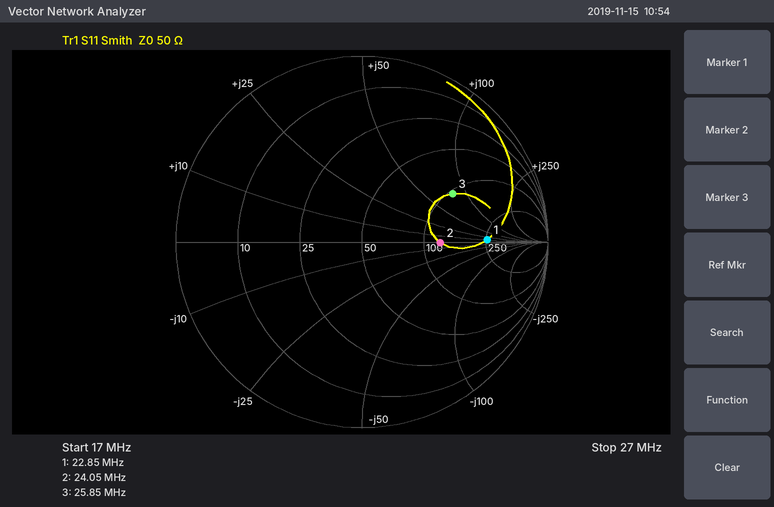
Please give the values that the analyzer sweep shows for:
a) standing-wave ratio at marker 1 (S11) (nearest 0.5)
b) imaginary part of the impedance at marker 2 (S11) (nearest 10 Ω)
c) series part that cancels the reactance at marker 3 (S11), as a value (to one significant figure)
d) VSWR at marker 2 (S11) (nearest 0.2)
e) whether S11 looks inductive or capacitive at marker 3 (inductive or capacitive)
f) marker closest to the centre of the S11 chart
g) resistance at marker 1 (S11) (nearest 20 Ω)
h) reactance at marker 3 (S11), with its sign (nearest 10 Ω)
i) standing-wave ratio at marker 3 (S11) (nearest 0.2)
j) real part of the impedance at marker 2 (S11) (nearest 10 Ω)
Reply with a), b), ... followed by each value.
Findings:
a) 5.0
b) 0 Ω
c) 80 pF
d) 2.4
e) inductive
f) marker 2
g) 260 Ω
h) +80 Ω
i) 3.4
j) 120 Ω
